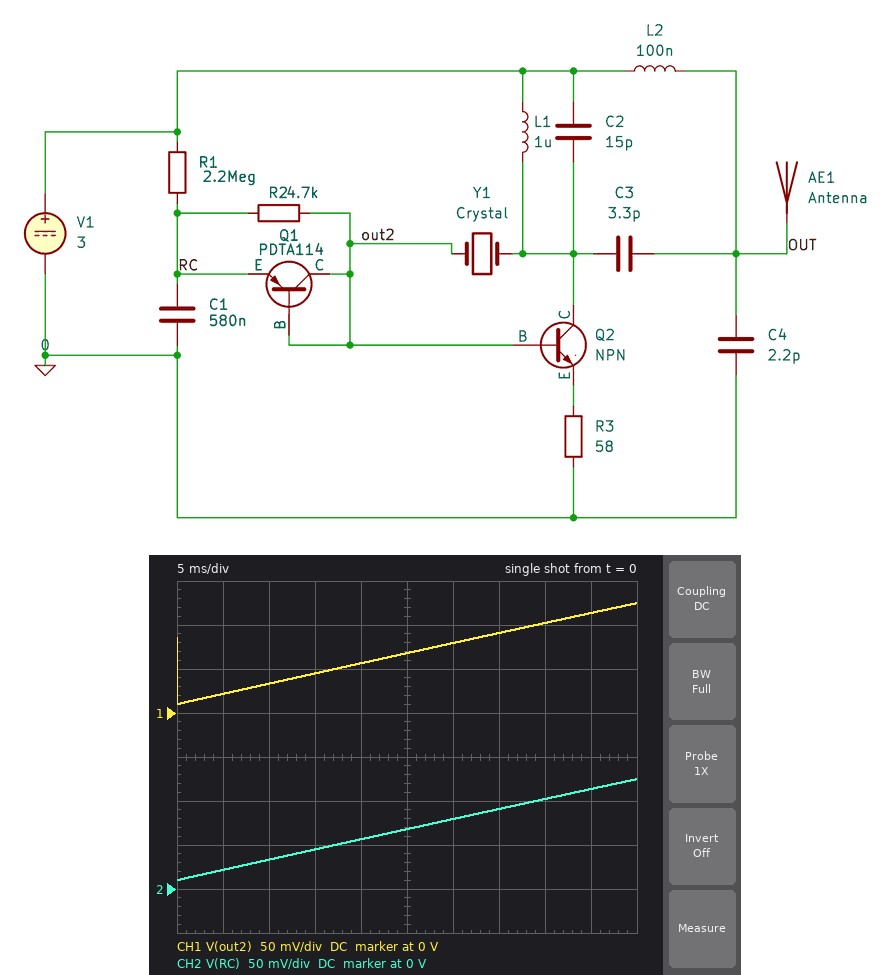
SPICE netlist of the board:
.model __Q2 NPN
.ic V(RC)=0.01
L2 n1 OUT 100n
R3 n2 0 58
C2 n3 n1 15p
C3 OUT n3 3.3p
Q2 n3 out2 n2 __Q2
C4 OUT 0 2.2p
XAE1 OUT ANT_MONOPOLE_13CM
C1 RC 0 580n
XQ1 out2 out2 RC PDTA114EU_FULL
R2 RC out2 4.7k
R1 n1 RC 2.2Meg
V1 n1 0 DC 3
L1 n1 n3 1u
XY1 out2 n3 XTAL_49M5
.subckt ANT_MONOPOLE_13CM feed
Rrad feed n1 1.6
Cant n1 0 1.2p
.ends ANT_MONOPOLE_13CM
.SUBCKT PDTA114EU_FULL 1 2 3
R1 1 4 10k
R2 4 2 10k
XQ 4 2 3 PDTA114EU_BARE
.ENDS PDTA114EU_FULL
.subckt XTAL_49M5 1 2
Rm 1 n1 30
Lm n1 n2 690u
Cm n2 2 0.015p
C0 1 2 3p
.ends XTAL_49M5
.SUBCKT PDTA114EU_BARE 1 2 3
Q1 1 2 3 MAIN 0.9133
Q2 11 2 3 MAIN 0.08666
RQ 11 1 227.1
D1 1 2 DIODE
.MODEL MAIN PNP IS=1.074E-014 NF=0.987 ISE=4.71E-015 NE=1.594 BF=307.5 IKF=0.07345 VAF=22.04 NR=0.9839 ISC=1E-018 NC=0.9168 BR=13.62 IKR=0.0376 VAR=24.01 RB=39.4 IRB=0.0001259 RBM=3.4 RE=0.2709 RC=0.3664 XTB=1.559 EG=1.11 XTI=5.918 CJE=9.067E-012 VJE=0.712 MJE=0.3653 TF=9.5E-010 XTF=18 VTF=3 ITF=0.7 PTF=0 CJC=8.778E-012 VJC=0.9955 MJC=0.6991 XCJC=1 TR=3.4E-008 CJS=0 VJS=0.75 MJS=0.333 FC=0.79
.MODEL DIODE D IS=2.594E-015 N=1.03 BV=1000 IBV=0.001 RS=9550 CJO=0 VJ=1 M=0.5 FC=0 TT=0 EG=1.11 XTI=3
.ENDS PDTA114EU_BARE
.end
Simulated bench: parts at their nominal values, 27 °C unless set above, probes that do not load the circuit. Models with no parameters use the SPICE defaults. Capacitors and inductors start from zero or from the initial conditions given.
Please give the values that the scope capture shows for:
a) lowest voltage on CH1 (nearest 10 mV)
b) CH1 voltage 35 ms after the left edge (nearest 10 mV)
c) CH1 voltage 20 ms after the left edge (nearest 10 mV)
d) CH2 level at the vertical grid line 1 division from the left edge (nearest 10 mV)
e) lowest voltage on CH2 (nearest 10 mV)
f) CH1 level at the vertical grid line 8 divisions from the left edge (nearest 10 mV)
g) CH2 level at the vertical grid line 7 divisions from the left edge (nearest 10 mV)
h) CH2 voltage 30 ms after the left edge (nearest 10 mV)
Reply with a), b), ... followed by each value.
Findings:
a) 10 mV
b) 90 mV
c) 60 mV
d) 20 mV
e) 10 mV
f) 100 mV
g) 90 mV
h) 80 mV
